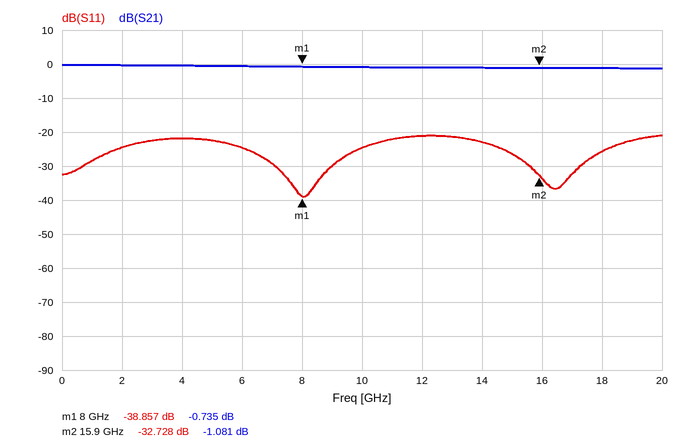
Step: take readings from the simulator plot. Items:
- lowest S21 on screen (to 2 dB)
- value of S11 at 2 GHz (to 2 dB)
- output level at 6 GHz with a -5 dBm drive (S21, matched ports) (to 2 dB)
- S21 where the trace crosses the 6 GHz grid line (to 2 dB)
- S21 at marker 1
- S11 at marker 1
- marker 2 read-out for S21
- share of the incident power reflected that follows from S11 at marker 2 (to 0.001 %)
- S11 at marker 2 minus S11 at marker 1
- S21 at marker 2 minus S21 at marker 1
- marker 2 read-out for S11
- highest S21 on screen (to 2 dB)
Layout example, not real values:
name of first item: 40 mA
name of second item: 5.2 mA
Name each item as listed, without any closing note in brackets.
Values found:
lowest S21 on screen: -2 dB
value of S11 at 2 GHz: -24 dB
output level at 6 GHz with a -5 dBm drive (S21, matched ports): -6 dBm
S21 where the trace crosses the 6 GHz grid line: 0 dB
S21 at marker 1: -0.735 dB
S11 at marker 1: -38.857 dB
marker 2 read-out for S21: -1.081 dB
share of the incident power reflected that follows from S11 at marker 2: 0.053 %
S11 at marker 2 minus S11 at marker 1: 6.129 dB
S21 at marker 2 minus S21 at marker 1: -0.346 dB
marker 2 read-out for S11: -32.728 dB
highest S21 on screen: 0 dB
